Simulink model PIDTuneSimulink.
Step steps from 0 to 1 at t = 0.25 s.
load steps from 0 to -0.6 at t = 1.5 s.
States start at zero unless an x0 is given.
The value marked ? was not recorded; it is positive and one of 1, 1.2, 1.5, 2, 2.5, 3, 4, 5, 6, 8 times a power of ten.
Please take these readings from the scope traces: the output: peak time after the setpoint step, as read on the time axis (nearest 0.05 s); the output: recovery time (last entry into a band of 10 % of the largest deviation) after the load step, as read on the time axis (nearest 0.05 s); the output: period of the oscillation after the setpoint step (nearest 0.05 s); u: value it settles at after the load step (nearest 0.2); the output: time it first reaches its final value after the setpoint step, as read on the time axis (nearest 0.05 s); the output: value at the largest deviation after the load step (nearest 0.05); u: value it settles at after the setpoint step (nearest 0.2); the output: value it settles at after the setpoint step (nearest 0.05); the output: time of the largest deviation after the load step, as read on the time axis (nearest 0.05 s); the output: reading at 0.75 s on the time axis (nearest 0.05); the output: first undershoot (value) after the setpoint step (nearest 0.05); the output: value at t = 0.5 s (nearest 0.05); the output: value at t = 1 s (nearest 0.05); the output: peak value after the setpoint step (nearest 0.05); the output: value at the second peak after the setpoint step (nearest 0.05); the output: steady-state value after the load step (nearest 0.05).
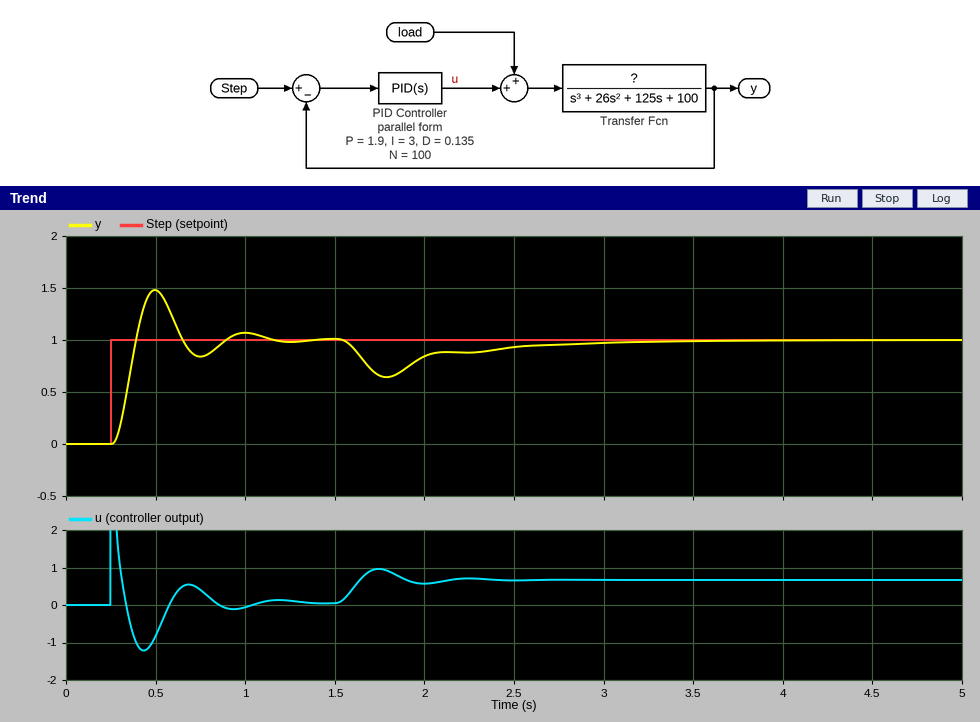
0.50 s
2.90 s
0.50 s
0.6
0.40 s
0.65
0.0
1.00
1.80 s
0.85
0.85
1.50
1.05
1.50
1.05
1.00
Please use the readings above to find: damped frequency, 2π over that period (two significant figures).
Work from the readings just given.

13 rad/s
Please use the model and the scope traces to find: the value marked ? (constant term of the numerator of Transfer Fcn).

1500
